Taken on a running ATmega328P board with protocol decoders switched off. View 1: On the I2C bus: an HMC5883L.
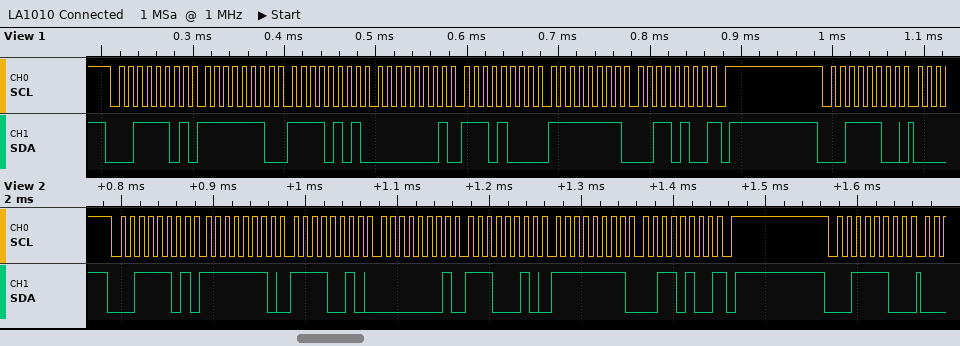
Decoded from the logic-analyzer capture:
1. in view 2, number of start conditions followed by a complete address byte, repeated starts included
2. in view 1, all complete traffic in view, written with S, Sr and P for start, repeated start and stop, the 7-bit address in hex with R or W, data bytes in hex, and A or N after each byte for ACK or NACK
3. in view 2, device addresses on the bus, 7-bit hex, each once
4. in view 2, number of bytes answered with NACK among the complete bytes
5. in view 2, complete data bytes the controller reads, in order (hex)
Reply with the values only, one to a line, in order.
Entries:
2
S 1ER A FE A F5 A 01 A E8 A FF A 34 N P S 1EW A
0x1E
1
FE F2 01 E2 FF 34
